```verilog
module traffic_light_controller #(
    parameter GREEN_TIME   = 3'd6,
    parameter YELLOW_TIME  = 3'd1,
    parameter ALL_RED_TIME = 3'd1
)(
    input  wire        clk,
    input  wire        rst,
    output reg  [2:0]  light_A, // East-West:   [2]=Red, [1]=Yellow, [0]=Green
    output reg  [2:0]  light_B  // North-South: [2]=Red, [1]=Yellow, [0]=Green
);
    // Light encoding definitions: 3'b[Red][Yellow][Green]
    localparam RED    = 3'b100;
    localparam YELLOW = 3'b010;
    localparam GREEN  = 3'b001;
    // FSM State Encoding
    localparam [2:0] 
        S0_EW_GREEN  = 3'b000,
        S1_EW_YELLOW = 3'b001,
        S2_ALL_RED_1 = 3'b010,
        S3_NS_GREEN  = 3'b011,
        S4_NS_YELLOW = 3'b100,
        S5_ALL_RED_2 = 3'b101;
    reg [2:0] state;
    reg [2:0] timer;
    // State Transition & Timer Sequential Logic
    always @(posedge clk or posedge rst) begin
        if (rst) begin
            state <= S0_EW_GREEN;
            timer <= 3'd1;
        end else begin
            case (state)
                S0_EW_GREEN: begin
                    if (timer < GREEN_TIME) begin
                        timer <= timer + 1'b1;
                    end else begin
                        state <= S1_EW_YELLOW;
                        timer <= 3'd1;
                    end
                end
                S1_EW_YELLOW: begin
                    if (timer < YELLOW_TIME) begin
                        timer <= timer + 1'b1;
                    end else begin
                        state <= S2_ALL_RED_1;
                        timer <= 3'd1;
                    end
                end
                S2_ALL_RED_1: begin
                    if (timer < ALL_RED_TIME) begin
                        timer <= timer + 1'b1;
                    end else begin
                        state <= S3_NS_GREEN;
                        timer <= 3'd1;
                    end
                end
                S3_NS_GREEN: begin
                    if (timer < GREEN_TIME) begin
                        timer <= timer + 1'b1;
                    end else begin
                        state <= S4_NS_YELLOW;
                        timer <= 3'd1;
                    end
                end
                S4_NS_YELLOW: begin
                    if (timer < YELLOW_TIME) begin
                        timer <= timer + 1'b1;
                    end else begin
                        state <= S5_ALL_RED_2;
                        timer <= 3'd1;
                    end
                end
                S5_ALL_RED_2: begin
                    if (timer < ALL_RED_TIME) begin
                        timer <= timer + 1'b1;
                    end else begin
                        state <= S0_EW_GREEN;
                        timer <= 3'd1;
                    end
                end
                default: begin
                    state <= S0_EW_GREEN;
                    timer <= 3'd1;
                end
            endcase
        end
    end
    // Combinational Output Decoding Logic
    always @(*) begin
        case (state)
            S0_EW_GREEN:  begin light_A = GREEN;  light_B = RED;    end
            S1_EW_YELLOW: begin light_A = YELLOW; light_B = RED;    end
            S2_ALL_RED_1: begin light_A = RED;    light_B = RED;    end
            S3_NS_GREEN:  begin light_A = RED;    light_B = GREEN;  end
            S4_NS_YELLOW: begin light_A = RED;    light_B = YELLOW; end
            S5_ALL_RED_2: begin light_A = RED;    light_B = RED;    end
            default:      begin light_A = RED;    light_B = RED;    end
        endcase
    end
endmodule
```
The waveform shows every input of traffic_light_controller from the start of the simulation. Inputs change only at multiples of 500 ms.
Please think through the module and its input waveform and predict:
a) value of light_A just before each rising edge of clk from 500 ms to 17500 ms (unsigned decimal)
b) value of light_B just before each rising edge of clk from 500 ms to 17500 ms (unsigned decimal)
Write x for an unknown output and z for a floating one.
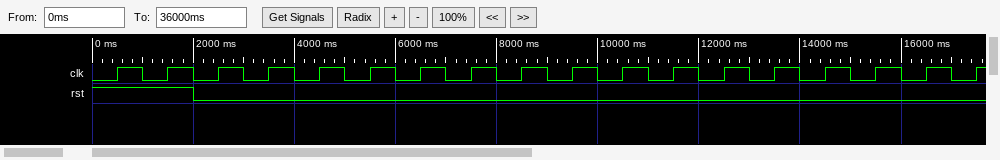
1, 1, 1, 1, 1, 1, 1, 1, 2, 4, 4, 4, 4, 4, 4, 4, 4, 4
4, 4, 4, 4, 4, 4, 4, 4, 4, 4, 1, 1, 1, 1, 1, 1, 2, 4
